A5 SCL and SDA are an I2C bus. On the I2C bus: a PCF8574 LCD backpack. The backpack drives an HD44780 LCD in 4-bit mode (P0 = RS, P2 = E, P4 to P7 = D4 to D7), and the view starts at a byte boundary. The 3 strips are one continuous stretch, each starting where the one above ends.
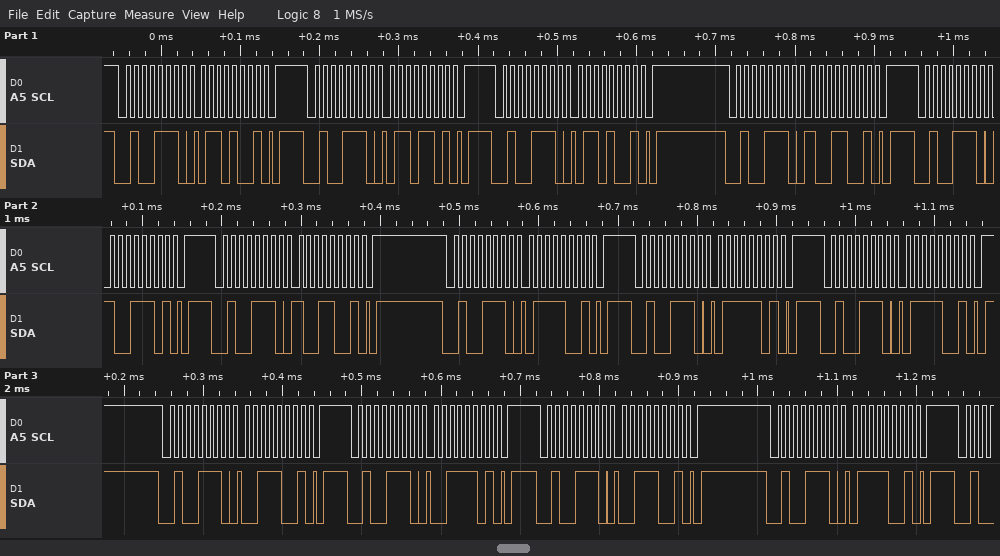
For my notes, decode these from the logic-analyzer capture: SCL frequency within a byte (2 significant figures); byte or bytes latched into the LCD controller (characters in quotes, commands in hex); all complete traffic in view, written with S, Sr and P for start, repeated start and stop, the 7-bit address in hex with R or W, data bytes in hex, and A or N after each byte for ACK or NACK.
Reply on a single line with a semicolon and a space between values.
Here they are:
100 kHz; 'i' 's'; S 27W A 69 A P S 27W A 6D A P S 27W A 69 A P S 27W A 99 A P S 27W A 9D A P S 27W A 99 A P S 27W A 79 A P S 27W A 7D A P S 27W A 79 A P S 27W A 39 A P S 27W A 3D A P S 27W A 39 A P S 27W A 79 A P
